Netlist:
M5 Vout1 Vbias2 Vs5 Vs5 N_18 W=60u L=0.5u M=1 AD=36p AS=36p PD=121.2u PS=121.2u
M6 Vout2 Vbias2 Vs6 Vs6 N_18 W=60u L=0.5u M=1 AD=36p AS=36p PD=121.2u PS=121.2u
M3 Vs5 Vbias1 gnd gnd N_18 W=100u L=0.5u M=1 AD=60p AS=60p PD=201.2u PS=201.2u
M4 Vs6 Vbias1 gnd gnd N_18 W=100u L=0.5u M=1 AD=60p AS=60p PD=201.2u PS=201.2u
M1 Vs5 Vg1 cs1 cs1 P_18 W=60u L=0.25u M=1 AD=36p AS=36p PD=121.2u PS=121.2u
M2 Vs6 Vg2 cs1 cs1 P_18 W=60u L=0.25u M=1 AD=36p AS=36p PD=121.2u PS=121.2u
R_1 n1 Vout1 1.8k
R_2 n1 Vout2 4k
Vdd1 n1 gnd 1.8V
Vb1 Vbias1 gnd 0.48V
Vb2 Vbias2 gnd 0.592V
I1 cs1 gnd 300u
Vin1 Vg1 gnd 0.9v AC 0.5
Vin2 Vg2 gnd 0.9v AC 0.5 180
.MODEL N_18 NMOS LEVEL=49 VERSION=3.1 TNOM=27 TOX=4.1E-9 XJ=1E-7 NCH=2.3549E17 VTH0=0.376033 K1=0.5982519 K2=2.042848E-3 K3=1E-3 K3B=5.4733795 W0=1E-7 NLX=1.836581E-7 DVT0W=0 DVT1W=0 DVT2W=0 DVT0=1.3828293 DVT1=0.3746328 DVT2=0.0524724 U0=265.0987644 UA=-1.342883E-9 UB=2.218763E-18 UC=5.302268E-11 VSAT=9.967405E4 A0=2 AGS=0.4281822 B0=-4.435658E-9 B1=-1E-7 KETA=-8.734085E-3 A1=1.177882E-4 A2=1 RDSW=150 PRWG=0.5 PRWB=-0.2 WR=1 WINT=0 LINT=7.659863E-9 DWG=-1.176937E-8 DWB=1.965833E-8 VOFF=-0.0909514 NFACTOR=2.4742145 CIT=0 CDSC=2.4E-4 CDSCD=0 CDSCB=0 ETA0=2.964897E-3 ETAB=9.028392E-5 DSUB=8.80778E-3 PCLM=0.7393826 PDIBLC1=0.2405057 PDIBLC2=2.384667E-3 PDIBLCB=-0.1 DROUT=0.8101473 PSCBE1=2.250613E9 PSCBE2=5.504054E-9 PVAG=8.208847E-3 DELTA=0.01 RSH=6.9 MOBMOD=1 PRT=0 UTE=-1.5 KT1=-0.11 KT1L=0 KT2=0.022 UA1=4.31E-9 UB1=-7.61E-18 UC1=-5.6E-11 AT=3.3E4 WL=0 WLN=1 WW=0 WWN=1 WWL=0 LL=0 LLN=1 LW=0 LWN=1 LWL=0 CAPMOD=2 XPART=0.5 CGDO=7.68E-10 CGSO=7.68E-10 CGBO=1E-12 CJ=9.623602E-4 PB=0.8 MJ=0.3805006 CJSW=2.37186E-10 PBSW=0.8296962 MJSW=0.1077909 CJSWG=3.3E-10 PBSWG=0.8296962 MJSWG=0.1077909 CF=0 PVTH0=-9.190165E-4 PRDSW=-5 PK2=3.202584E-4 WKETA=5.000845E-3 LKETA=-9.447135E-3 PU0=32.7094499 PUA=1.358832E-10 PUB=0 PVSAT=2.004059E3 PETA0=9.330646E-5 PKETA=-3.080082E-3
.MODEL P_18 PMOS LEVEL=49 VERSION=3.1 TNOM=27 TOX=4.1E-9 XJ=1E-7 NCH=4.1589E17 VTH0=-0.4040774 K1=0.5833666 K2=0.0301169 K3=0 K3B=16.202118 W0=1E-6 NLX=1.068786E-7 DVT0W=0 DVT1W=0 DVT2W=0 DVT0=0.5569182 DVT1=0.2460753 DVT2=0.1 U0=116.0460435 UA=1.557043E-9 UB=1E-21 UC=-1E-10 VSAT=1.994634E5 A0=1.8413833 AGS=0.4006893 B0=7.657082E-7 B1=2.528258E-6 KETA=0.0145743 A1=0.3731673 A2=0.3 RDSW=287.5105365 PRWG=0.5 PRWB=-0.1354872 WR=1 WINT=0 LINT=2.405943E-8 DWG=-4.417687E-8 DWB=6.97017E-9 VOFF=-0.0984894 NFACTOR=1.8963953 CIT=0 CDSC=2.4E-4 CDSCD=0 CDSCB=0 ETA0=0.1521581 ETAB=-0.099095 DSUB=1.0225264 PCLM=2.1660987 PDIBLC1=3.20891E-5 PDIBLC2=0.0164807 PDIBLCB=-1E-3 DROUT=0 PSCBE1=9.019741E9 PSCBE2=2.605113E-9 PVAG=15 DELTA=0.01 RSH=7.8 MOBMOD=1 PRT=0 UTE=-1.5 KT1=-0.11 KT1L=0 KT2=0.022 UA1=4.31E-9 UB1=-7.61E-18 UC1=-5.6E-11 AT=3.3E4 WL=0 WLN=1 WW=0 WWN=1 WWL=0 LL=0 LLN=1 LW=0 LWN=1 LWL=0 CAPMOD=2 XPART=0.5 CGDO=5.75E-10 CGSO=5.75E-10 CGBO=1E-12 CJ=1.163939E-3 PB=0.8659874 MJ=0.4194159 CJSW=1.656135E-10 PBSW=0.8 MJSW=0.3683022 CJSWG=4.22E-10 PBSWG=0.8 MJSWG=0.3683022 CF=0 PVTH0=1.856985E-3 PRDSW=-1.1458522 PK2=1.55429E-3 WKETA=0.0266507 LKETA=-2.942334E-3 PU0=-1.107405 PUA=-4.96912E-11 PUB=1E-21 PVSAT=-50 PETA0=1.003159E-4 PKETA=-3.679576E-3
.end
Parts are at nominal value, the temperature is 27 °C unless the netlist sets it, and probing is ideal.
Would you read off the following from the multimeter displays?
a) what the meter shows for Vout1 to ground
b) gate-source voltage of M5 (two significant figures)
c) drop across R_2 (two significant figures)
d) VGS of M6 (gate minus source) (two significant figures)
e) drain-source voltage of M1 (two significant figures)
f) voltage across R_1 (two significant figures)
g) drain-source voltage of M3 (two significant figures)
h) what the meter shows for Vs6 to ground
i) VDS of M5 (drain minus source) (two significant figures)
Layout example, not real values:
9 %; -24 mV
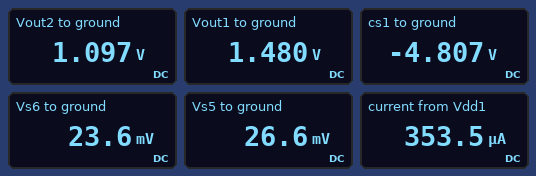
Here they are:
1.480 V; 570 mV; 700 mV; 570 mV; 4.8 V; 320 mV; 27 mV; 23.6 mV; 1.5 V
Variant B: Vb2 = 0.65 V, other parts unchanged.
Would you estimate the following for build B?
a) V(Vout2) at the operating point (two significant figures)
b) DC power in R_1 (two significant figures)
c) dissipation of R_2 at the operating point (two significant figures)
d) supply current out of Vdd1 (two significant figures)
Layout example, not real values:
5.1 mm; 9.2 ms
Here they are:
1.0 V; 69 µW; 150 µW; 390 µA
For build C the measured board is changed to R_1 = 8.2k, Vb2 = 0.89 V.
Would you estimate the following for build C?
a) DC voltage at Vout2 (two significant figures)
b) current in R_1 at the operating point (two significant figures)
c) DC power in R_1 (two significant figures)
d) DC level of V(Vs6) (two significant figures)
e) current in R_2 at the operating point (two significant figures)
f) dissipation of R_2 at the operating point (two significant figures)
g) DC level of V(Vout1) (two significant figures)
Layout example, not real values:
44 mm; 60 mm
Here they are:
970 mV; 200 µA; 330 µW; 310 mV; 210 µA; 170 µW; 160 mV
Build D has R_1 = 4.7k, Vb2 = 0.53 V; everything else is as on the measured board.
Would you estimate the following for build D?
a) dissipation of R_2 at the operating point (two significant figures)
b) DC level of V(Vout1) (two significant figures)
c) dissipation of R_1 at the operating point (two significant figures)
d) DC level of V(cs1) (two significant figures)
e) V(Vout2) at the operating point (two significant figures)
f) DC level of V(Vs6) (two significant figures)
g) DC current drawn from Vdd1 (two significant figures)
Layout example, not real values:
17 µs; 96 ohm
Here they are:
63 µW; 1.2 V; 73 µW; -4.8 V; 1.3 V; -15 mV; 250 µA
